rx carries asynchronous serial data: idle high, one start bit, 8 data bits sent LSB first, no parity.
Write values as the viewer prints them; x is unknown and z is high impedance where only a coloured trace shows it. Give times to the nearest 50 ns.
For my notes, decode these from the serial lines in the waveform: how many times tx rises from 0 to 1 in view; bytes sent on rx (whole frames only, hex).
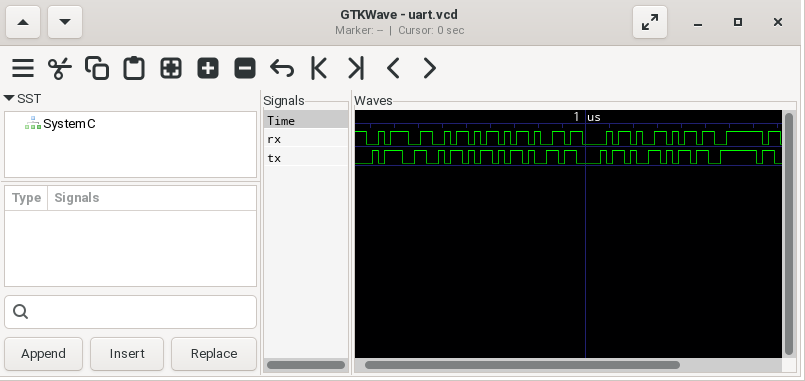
21
3A, 5A, 2D, 43, 59, F3
